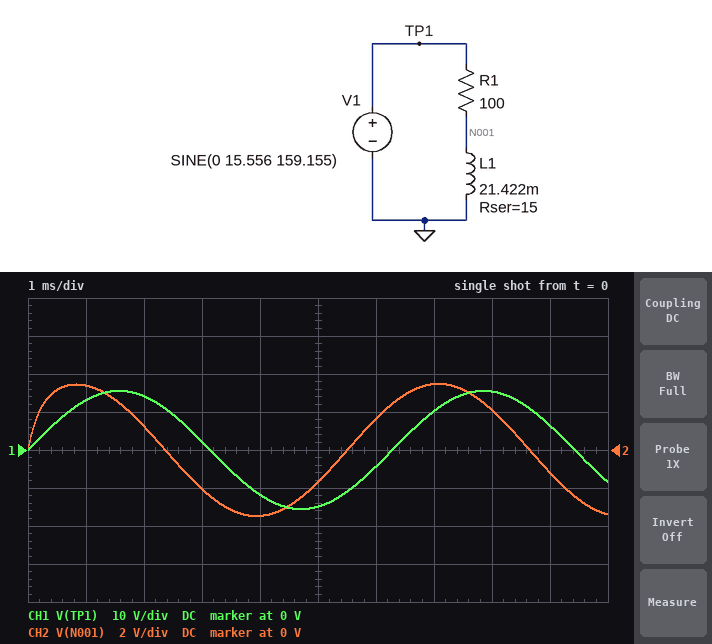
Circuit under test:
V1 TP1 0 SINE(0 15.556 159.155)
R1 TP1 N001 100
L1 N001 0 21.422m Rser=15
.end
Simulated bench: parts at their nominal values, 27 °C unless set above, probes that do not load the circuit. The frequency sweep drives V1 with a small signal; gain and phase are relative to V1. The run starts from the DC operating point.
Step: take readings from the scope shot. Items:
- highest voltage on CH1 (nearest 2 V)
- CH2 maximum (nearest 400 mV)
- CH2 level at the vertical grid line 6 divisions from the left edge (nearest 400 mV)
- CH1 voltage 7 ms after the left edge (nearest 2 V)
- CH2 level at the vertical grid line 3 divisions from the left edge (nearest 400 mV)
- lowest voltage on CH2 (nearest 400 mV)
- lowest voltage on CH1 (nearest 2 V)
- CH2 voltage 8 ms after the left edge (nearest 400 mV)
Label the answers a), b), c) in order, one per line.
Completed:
a) 16 V
b) 3.6 V
c) 1.6 V
d) 10 V
e) -2.0 V
f) -3.6 V
g) -16 V
h) 2.0 V
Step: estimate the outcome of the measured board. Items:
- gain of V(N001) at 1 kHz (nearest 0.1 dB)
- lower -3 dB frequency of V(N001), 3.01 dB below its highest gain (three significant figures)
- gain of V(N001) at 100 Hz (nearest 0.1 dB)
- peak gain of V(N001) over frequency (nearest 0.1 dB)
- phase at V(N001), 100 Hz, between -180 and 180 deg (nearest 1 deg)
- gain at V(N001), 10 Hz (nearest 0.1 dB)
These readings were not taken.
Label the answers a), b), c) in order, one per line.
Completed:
a) -2.3 dB
b) 840 Hz
c) -15.2 dB
d) 0 dB
e) 35 deg
f) -17.7 dB
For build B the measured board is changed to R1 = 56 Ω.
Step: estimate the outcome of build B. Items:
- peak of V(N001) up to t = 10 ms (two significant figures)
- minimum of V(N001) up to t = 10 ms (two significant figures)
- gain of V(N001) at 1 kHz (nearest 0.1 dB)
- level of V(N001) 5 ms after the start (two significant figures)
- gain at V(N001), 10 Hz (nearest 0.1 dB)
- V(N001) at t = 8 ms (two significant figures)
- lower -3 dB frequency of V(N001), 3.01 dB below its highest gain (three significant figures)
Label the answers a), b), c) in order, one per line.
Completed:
a) 5.5 V
b) -5.5 V
c) -1.0 dB
d) -3.2 V
e) -13.5 dB
f) 3.8 V
g) 503 Hz
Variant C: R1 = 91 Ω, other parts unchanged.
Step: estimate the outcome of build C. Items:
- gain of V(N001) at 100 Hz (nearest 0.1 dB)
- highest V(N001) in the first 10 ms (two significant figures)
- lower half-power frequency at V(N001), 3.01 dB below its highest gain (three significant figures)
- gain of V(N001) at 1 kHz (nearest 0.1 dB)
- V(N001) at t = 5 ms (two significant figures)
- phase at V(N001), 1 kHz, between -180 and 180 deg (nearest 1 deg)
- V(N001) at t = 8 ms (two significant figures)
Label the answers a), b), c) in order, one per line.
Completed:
a) -14.5 dB
b) 3.8 V
c) 772 Hz
d) -2.0 dB
e) -1.9 V
f) 32 deg
g) 2.3 V
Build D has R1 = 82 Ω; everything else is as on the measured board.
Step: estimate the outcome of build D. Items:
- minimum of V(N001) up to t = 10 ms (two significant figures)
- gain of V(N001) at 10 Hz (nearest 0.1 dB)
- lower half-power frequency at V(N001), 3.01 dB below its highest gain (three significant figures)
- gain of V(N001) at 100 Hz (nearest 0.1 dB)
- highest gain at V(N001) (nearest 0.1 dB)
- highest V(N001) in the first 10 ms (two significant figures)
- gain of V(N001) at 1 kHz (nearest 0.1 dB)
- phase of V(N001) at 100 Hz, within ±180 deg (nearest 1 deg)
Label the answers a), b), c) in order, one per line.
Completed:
a) -4.1 V
b) -16.2 dB
c) 703 Hz
d) -13.7 dB
e) 0 dB
f) 4.1 V
g) -1.8 dB
h) 34 deg
